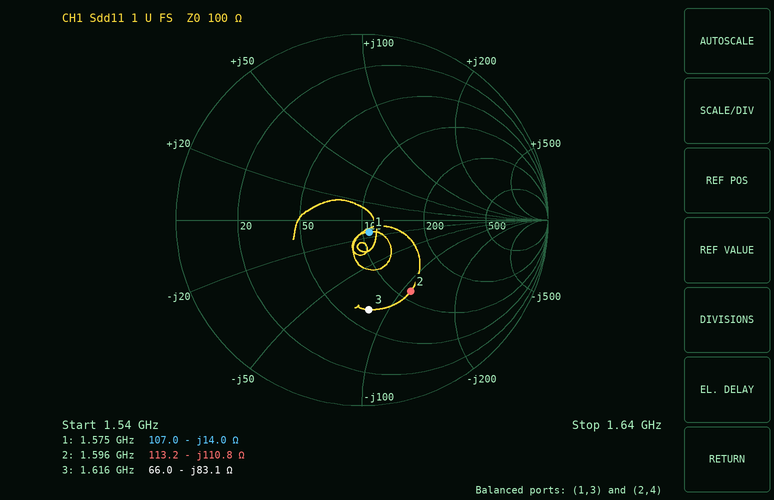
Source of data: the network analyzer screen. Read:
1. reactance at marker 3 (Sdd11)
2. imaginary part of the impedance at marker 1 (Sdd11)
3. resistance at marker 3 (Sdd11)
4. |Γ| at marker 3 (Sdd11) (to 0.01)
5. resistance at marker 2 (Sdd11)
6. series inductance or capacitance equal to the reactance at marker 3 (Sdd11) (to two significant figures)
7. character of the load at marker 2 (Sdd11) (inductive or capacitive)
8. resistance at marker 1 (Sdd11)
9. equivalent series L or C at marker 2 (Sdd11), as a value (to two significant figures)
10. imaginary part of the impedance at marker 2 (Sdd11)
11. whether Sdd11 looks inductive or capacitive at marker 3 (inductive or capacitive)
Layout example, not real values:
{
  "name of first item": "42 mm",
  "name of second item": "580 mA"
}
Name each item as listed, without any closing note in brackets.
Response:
{
  "reactance at marker 3": "-83.1 Ω",
  "imaginary part of the impedance at marker 1": "-14.0 Ω",
  "resistance at marker 3": "66.0 Ω",
  "|Γ| at marker 3 (Sdd11)": "0.48",
  "resistance at marker 2": "113.2 Ω",
  "series inductance or capacitance equal to the reactance at marker 3 (Sdd11)": "1.2 pF",
  "character of the load at marker 2 (Sdd11)": "capacitive",
  "resistance at marker 1": "107.0 Ω",
  "equivalent series L or C at marker 2 (Sdd11), as a value": "900 fF",
  "imaginary part of the impedance at marker 2": "-110.8 Ω",
  "whether Sdd11 looks inductive or capacitive at marker 3": "capacitive"
}
